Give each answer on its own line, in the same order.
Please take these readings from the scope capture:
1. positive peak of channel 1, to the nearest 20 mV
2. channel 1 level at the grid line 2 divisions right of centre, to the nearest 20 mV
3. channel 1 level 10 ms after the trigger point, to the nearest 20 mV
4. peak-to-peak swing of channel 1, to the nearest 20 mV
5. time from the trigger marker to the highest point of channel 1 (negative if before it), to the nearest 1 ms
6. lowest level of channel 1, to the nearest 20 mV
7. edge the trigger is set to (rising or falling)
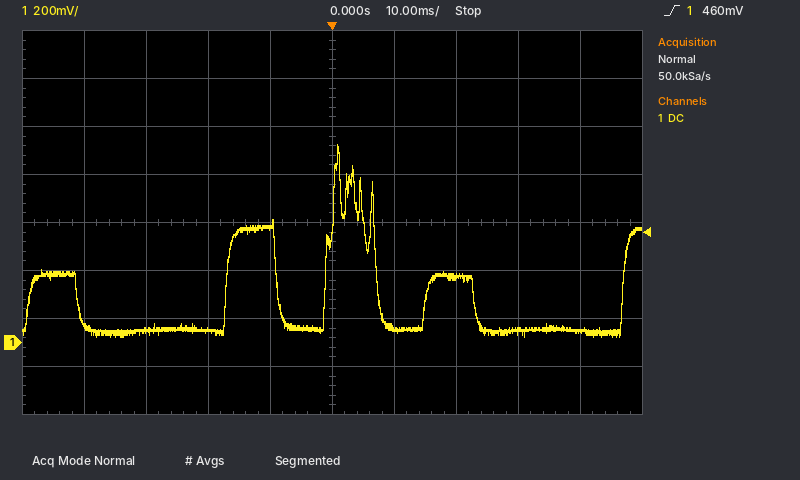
820 mV
280 mV
60 mV
800 mV
+1 ms
20 mV
rising
